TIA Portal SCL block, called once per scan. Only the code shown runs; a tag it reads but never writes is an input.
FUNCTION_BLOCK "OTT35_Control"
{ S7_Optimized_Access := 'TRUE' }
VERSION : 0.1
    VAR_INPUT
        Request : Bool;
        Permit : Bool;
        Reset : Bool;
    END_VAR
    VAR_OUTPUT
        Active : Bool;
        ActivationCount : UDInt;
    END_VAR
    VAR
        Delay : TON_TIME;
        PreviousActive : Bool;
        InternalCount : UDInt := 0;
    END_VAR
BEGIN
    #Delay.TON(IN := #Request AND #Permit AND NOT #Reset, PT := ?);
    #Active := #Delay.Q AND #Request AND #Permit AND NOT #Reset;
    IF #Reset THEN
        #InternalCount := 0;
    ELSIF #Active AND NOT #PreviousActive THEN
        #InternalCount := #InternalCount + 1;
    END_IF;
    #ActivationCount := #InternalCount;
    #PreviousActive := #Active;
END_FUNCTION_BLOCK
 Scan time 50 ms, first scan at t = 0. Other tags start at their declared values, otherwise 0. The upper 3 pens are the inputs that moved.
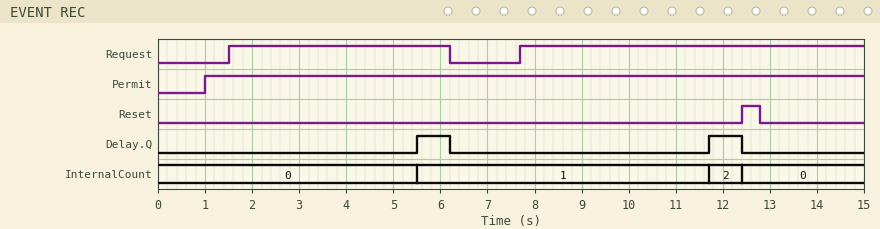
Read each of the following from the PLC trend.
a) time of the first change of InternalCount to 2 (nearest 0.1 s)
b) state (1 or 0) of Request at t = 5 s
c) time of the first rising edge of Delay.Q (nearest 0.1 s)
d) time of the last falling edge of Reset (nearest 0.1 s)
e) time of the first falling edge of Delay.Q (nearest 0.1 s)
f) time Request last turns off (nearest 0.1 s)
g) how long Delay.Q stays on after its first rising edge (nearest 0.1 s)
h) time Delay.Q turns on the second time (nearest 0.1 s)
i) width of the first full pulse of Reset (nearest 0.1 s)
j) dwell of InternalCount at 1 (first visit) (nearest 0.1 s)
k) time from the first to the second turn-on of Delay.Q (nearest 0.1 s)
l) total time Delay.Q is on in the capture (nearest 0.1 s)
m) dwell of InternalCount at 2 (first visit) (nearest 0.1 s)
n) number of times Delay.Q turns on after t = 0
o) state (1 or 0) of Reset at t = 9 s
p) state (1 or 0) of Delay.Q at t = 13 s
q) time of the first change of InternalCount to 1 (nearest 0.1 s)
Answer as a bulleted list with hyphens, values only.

- 11.7 s
- 1
- 5.5 s
- 12.8 s
- 6.2 s
- 6.2 s
- 0.7 s
- 11.7 s
- 0.4 s
- 6.2 s
- 6.2 s
- 1.4 s
- 0.7 s
- 2
- 0
- 0
- 5.5 s
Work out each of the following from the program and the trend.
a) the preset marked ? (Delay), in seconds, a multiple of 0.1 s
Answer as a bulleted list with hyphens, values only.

- 4.0 s
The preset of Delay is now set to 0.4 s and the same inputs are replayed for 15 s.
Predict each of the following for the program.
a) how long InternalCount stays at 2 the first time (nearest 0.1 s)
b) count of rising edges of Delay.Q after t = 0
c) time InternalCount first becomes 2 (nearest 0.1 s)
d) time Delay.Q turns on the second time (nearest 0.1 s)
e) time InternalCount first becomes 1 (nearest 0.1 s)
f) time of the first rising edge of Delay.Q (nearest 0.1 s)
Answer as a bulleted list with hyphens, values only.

- 4.3 s
- 3
- 8.1 s
- 8.1 s
- 1.9 s
- 1.9 s
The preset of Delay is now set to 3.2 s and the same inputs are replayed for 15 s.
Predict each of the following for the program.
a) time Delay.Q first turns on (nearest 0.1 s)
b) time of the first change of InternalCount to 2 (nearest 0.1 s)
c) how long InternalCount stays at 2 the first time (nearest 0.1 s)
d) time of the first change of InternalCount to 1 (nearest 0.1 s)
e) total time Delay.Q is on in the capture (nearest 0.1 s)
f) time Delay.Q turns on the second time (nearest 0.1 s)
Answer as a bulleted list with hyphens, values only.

- 4.7 s
- 10.9 s
- 1.5 s
- 4.7 s
- 3.0 s
- 10.9 s
